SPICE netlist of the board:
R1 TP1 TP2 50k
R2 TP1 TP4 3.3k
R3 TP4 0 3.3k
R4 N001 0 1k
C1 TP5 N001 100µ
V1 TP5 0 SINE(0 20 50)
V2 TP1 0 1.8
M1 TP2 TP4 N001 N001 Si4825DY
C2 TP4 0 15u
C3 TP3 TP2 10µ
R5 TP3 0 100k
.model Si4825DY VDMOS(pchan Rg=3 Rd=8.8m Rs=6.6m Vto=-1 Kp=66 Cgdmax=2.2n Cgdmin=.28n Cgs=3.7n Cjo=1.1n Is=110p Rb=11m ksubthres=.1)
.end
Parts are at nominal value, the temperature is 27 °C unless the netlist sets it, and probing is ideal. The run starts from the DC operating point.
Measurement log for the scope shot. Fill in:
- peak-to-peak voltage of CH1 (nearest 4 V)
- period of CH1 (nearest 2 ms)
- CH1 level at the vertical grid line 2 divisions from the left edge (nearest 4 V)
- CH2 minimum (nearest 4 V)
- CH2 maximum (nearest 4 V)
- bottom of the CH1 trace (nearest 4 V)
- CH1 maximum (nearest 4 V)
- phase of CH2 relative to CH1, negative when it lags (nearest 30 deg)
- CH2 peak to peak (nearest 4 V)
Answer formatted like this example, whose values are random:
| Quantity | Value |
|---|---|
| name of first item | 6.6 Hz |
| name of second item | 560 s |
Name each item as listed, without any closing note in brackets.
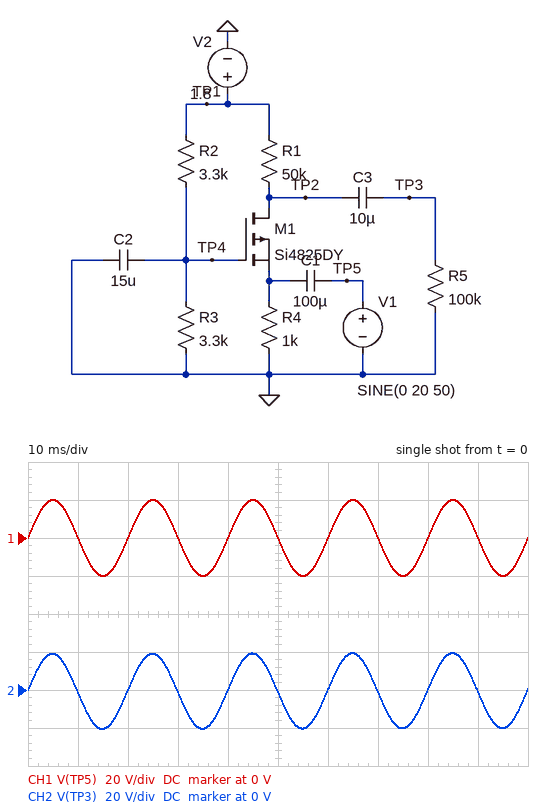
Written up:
| Quantity | Value |
|---|---|
| peak-to-peak voltage of CH1 | 40 V |
| period of CH1 | 20 ms |
| CH1 level at the vertical grid line 2 divisions from the left edge | 0 V |
| CH2 minimum | -20 V |
| CH2 maximum | 20 V |
| bottom of the CH1 trace | -20 V |
| CH1 maximum | 20 V |
| phase of CH2 relative to CH1, negative when it lags | 0 deg |
| CH2 peak to peak | 40 V |
